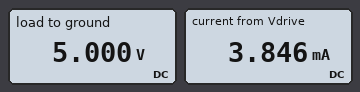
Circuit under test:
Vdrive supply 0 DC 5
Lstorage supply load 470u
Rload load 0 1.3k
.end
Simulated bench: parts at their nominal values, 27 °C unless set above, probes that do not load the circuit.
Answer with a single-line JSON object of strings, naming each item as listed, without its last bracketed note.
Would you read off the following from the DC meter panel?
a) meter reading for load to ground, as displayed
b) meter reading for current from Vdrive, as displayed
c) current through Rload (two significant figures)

{"meter reading for load to ground, as displayed": "5.000 V", "meter reading for current from Vdrive, as displayed": "3.846 mA", "current through Rload": "3.8 mA"}
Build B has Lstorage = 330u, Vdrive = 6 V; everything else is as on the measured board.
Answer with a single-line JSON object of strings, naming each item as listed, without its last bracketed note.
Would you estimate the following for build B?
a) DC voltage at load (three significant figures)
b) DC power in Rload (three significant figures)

{"DC voltage at load": "6.00 V", "DC power in Rload": "27.7 mW"}
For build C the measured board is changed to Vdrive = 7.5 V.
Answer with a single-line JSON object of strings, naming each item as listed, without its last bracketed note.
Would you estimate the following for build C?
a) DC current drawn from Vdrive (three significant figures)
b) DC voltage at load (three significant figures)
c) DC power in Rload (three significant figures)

{"DC current drawn from Vdrive": "5.77 mA", "DC voltage at load": "7.50 V", "DC power in Rload": "43.3 mW"}
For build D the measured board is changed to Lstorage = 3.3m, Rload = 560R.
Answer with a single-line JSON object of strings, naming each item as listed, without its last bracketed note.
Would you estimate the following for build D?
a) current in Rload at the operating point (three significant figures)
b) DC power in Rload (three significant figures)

{"current in Rload at the operating point": "8.93 mA", "DC power in Rload": "44.6 mW"}
